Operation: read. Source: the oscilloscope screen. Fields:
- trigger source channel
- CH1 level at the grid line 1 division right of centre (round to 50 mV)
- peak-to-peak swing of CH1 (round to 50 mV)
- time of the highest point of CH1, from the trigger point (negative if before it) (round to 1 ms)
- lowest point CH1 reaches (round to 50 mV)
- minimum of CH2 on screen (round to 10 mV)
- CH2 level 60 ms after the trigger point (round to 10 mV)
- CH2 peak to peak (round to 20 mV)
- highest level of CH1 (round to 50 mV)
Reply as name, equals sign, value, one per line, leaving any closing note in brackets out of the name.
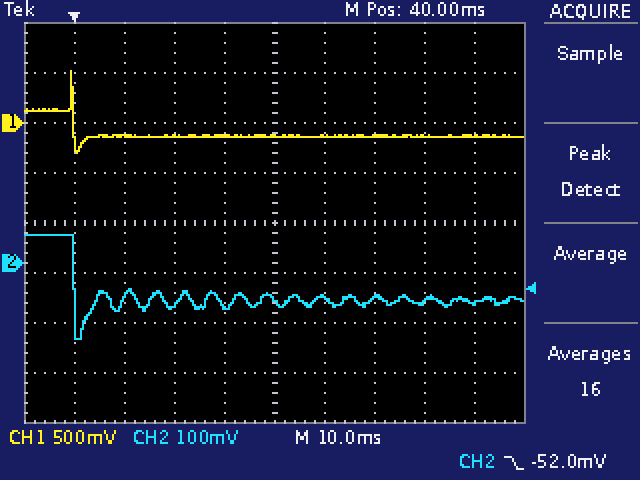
trigger source channel = CH2
CH1 level at the grid line 1 division right of centre = -150 mV
peak-to-peak swing of CH1 = 800 mV
time of the highest point of CH1, from the trigger point (negative if before it) = -1 ms
lowest point CH1 reaches = -300 mV
minimum of CH2 on screen = -150 mV
CH2 level 60 ms after the trigger point = -70 mV
CH2 peak to peak = 200 mV
highest level of CH1 = 500 mV
